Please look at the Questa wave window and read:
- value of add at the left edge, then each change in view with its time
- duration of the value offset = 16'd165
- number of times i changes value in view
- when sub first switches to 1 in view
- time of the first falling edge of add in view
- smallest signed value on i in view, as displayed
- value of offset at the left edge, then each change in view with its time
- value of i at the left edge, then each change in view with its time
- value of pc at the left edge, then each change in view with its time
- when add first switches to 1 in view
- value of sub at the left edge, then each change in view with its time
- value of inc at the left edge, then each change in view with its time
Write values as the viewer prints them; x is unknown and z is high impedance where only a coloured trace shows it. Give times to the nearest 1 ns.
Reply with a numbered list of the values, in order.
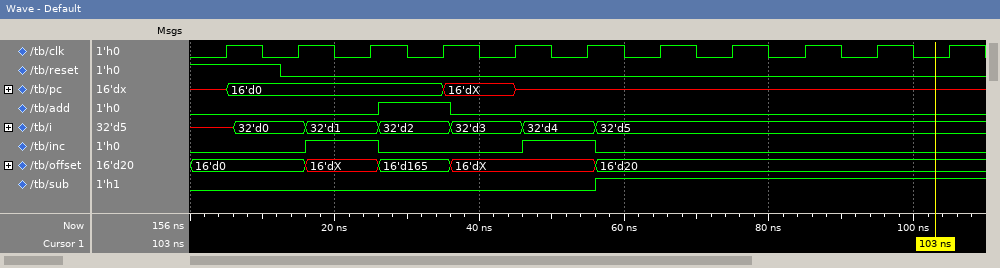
1. 0, 1 at 26 ns, 0 at 36 ns
2. 10 ns
3. 6
4. 56 ns
5. 36 ns
6. 32'd0
7. 16'd0, 16'dX at 16 ns, 16'd165 at 26 ns, 16'dX at 36 ns, 16'd20 at 56 ns
8. x, 32'd0 at 6 ns, 32'd1 at 16 ns, 32'd2 at 26 ns, 32'd3 at 36 ns, 32'd4 at 46 ns, 32'd5 at 56 ns
9. x, 16'd0 at 5 ns, 16'dX at 35 ns, x at 45 ns
10. 26 ns
11. 0, 1 at 56 ns
12. 0, 1 at 16 ns, 0 at 26 ns, 1 at 46 ns, 0 at 56 ns
